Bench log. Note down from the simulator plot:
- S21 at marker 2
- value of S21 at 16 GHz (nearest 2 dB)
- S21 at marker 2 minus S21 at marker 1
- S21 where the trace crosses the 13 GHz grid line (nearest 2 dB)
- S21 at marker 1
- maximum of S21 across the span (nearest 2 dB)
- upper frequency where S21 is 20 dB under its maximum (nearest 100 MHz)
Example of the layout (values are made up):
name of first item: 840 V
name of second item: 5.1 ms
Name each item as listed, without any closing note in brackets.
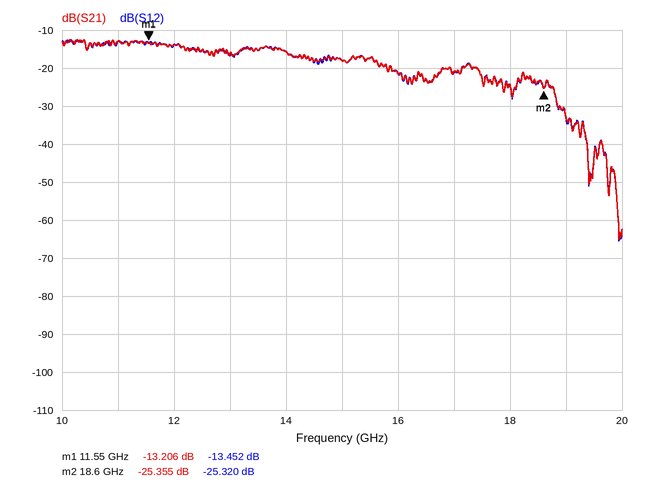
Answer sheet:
S21 at marker 2: -25.355 dB
value of S21 at 16 GHz: -22 dB
S21 at marker 2 minus S21 at marker 1: -12.149 dB
S21 where the trace crosses the 13 GHz grid line: -16 dB
S21 at marker 1: -13.206 dB
maximum of S21 across the span: -12 dB
upper frequency where S21 is 20 dB under its maximum: 19.0 GHz
